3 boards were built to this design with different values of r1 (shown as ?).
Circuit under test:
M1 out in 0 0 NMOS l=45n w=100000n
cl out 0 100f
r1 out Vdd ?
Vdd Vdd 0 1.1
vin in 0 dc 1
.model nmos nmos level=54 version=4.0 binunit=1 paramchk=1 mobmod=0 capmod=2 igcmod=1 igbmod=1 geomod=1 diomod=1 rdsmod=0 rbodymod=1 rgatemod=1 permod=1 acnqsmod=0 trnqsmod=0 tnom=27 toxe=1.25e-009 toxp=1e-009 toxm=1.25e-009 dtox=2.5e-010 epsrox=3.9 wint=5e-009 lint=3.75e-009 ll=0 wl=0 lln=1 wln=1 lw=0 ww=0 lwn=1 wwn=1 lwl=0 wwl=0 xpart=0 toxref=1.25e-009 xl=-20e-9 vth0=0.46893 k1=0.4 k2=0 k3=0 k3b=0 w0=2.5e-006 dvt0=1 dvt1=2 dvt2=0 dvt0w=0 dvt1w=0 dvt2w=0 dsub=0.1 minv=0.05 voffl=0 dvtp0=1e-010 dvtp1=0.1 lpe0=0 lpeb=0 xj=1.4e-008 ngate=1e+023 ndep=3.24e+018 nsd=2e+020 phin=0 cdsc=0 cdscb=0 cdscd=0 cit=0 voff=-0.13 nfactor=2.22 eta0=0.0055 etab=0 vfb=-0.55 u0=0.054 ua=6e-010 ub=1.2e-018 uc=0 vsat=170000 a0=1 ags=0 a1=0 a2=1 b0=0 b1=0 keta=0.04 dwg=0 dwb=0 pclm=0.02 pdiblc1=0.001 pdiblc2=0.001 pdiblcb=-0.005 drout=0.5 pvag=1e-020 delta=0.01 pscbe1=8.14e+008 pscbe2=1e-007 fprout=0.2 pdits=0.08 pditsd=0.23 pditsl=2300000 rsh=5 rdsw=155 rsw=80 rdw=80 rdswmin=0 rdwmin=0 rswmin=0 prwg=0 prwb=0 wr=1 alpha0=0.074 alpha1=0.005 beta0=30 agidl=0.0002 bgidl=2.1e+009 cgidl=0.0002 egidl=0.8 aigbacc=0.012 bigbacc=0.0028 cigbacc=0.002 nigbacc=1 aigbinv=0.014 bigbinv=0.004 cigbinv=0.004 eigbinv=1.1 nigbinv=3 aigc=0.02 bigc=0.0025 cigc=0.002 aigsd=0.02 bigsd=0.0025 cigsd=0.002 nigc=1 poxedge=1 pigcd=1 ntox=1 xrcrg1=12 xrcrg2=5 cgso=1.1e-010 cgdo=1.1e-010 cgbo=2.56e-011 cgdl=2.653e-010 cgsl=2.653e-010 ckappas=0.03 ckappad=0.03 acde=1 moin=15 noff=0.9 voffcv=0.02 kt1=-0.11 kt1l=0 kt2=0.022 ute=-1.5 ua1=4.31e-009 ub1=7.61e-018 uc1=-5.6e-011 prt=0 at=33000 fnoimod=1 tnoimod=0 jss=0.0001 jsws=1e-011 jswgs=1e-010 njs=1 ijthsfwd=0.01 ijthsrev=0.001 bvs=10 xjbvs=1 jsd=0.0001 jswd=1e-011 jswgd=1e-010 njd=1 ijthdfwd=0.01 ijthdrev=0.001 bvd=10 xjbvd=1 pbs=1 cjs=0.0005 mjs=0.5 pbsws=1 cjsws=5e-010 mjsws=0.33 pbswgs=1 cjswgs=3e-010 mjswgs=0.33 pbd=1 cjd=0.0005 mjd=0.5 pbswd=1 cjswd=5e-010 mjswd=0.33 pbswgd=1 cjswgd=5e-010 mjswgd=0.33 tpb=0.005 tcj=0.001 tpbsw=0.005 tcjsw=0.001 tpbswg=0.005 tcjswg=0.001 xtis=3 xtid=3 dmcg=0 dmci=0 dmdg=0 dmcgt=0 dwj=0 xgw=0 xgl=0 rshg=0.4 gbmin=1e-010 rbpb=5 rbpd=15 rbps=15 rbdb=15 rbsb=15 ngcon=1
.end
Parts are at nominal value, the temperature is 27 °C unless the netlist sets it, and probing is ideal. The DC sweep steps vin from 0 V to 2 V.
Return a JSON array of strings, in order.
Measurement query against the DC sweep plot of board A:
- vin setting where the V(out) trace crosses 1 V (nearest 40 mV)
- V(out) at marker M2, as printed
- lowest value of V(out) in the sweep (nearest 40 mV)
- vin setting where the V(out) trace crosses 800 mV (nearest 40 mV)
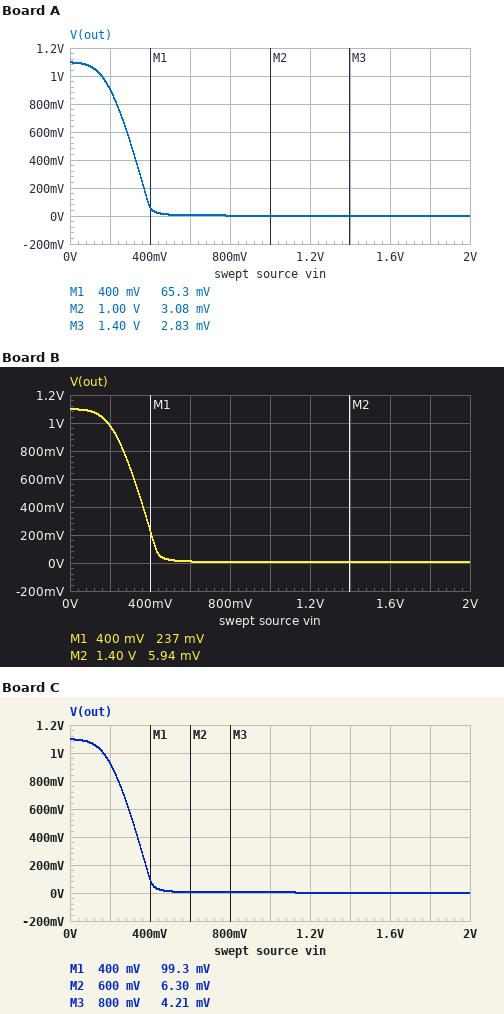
["160 mV", "3.08 mV", "0 V", "240 mV"]
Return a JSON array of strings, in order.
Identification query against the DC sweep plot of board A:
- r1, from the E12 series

["820 Ω"]
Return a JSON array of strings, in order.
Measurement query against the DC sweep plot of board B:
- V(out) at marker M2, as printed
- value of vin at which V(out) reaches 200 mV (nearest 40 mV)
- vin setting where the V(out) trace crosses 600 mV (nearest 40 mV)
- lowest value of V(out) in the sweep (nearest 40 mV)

["5.94 mV", "400 mV", "320 mV", "0 V"]
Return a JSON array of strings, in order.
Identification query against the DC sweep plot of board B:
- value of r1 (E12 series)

["390 Ω"]
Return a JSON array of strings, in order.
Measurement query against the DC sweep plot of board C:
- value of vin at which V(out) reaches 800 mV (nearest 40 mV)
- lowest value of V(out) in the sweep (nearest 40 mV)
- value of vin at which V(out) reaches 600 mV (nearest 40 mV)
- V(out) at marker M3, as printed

["240 mV", "0 V", "280 mV", "4.21 mV"]
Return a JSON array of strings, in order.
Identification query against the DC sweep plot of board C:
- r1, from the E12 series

["680 Ω"]
